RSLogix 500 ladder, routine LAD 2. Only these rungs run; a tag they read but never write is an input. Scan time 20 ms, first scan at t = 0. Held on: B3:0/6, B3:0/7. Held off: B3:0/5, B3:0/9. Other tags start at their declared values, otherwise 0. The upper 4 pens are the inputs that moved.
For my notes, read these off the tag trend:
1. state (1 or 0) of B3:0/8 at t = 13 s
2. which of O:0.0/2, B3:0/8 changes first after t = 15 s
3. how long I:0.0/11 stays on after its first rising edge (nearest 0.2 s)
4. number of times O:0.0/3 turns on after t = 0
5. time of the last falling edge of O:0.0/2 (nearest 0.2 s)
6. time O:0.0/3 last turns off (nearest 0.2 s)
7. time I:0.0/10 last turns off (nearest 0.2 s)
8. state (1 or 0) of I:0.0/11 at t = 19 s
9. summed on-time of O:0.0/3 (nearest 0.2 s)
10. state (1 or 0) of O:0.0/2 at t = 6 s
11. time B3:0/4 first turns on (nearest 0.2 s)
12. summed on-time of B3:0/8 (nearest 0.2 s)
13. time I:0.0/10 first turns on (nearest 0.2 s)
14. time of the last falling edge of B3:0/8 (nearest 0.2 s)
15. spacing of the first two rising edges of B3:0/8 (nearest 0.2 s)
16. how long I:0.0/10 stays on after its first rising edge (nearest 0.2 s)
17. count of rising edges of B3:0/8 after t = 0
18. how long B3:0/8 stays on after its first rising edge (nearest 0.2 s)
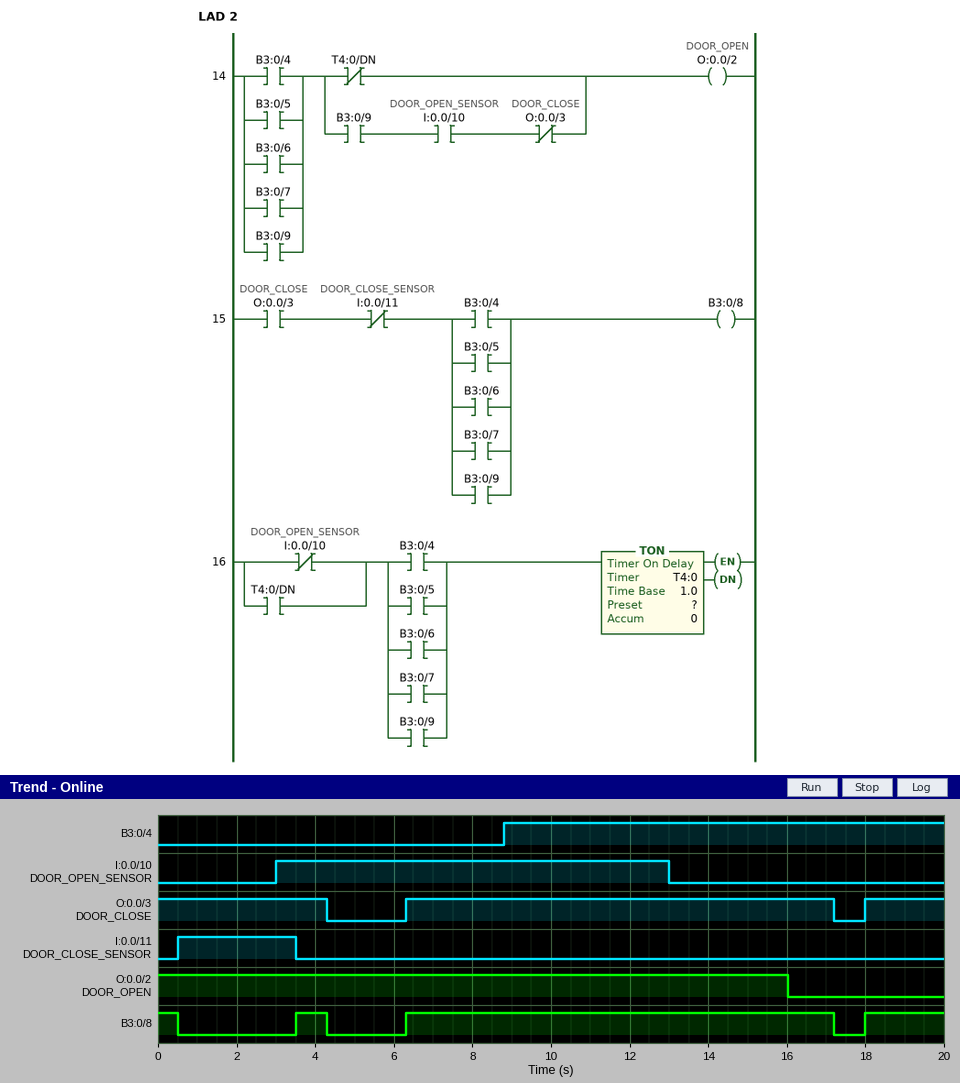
1
O:0.0/2
3.0 s
2
16.0 s
17.2 s
13.0 s
0
17.2 s
1
8.8 s
14.2 s
3.0 s
17.2 s
2.8 s
10.0 s
3
0.8 s
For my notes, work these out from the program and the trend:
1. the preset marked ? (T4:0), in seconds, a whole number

3 s
